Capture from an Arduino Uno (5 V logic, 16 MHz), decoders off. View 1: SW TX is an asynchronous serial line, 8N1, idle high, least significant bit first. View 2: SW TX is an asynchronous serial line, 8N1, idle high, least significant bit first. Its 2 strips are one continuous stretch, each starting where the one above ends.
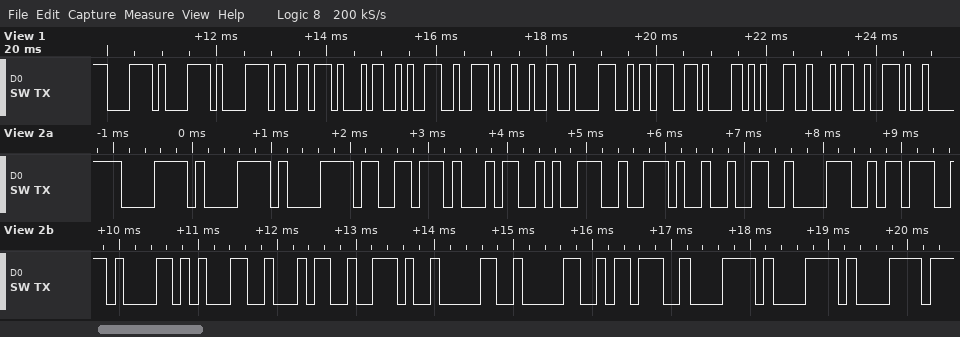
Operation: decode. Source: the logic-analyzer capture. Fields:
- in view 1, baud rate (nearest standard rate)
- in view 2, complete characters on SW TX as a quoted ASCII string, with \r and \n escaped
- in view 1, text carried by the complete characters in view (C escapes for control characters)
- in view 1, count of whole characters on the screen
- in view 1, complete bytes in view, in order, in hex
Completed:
9600 baud
"xxxv49.28;a14.00;xxx"
"xxxv49.28;a14."
14
78 78 78 76 34 39 2E 32 38 3B 61 31 34 2E
